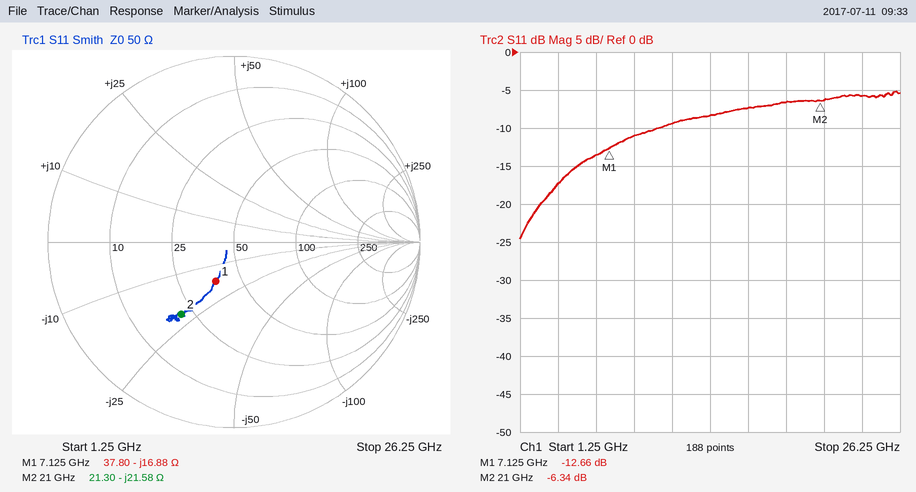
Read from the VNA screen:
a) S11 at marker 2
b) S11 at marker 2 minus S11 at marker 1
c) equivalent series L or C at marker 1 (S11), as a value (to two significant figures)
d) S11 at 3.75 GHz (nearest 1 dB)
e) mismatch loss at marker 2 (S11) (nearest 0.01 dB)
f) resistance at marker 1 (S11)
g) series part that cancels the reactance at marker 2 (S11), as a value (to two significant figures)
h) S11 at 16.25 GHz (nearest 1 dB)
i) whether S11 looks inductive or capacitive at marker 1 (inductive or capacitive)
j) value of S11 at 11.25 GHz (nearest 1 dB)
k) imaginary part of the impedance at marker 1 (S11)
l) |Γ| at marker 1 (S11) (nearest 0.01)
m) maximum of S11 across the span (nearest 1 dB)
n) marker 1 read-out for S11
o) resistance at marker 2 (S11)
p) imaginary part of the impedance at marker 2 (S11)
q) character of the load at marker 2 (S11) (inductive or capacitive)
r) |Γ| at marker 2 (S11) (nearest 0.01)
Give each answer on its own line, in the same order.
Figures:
-6.34 dB
6.32 dB
1.3 pF
-17 dB
1.15 dB
37.80 Ω
160 pH
-7 dB
capacitive
-9 dB
-16.88 Ω
0.23
-5 dB
-12.66 dB
21.30 Ω
-21.58 Ω
capacitive
0.48
